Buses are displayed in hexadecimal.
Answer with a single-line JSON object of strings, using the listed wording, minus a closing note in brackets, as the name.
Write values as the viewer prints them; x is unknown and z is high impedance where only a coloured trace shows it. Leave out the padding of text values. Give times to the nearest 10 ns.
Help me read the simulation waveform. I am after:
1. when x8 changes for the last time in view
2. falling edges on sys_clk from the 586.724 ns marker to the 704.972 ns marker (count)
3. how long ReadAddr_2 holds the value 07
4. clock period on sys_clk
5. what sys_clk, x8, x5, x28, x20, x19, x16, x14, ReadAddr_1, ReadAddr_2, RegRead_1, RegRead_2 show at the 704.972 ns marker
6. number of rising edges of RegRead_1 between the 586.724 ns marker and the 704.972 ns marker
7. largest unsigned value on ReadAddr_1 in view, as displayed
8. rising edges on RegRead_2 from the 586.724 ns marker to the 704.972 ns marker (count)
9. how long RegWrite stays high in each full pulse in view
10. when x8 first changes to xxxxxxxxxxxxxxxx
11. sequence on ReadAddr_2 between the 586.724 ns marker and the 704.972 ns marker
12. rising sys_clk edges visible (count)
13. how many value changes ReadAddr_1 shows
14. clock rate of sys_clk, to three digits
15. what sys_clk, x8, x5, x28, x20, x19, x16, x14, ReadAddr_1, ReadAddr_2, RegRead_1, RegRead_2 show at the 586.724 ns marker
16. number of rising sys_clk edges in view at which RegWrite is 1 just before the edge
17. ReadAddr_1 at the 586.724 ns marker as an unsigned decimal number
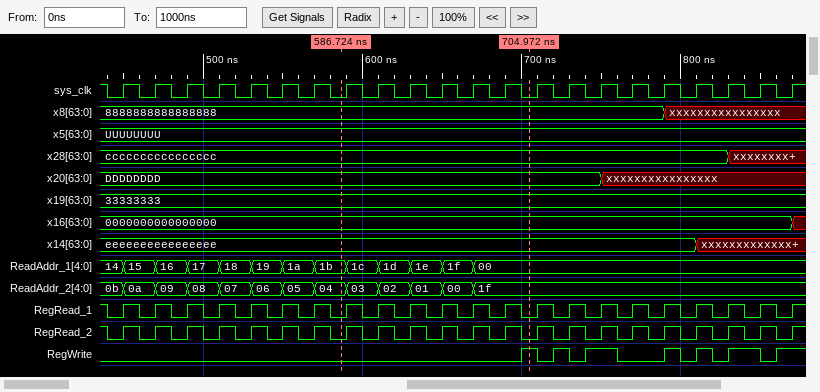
{"when x8 changes for the last time in view": "790 ns", "falling edges on sys_clk from the 586.724 ns marker to the 704.972 ns marker": "6", "how long ReadAddr_2 holds the value 07": "20 ns", "clock period on sys_clk": "20 ns", "what sys_clk, x8, x5, x28, x20, x19, x16, x14, ReadAddr_1, ReadAddr_2, RegRead_1, RegRead_2 show at the 704.972 ns marker": "sys_clk=0, x8=8888888888888888, x5=UUUUUUUU, x28=cccccccccccccccc, x20=DDDDDDDD, x19=33333333, x16=0000000000000000, x14=eeeeeeeeeeeeeeee, ReadAddr_1=00, ReadAddr_2=1f, RegRead_1=0, RegRead_2=0", "number of rising edges of RegRead_1 between the 586.724 ns marker and the 704.972 ns marker": "6", "largest unsigned value on ReadAddr_1 in view, as displayed": "1f", "rising edges on RegRead_2 from the 586.724 ns marker to the 704.972 ns marker": "6", "how long RegWrite stays high in each full pulse in view": "10 ns, 10 ns, 20 ns, 10 ns, 10 ns, 20 ns", "when x8 first changes to xxxxxxxxxxxxxxxx": "790 ns", "sequence on ReadAddr_2 between the 586.724 ns marker and the 704.972 ns marker": "04, 03, 02, 01, 00, 1f", "rising sys_clk edges visible": "22", "how many value changes ReadAddr_1 shows": "12", "clock rate of sys_clk, to three digits": "50.0 MHz", "what sys_clk, x8, x5, x28, x20, x19, x16, x14, ReadAddr_1, ReadAddr_2, RegRead_1, RegRead_2 show at the 586.724 ns marker": "sys_clk=0, x8=8888888888888888, x5=UUUUUUUU, x28=cccccccccccccccc, x20=DDDDDDDD, x19=33333333, x16=0000000000000000, x14=eeeeeeeeeeeeeeee, ReadAddr_1=1b, ReadAddr_2=04, RegRead_1=0, RegRead_2=0", "number of rising sys_clk edges in view at which RegWrite is 1 just before the edge": "5", "ReadAddr_1 at the 586.724 ns marker as an unsigned decimal number": "27"}
